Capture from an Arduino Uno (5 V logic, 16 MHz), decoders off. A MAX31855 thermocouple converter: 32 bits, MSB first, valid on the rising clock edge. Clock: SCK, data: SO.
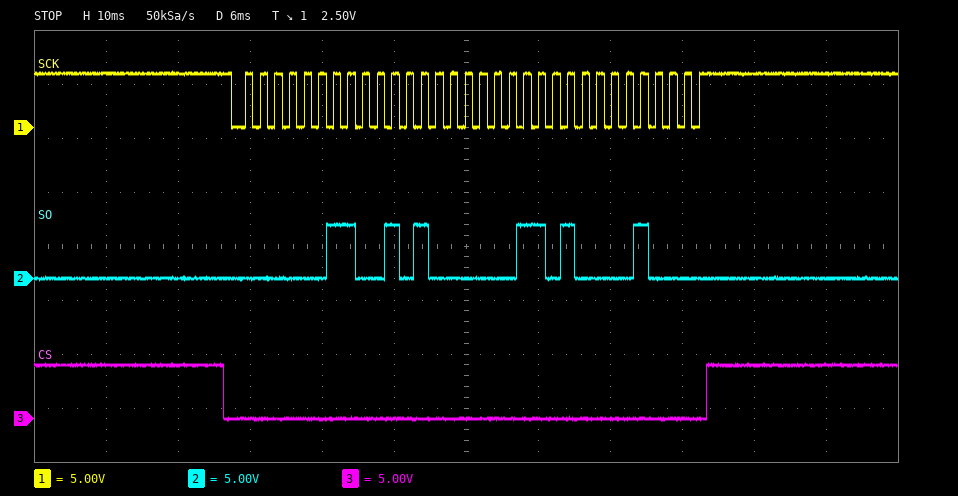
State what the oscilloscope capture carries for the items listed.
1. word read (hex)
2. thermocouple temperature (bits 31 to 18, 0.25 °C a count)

0x03281A10
50.50 °C
